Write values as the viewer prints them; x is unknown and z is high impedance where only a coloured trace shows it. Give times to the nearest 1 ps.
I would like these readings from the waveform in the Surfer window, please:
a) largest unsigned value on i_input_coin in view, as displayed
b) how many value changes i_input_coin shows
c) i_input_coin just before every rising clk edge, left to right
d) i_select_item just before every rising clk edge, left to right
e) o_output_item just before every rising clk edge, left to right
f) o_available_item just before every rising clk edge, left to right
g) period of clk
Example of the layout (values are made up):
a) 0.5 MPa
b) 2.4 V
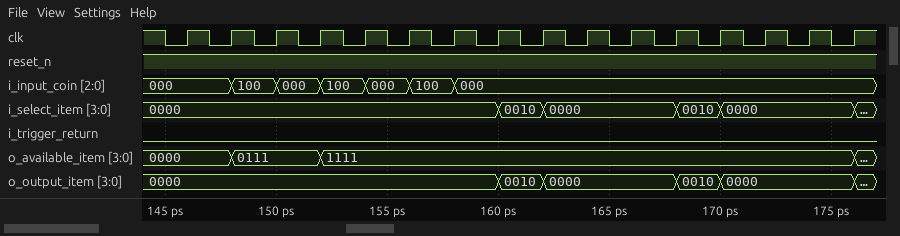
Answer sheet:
a) 100
b) 6
c) 000, 000, 100, 000, 100, 000, 100, 000, 000, 000, 000, 000, 000, 000, 000, 000
d) 0000, 0000, 0000, 0000, 0000, 0000, 0000, 0000, 0010, 0000, 0000, 0000, 0010, 0000, 0000, 0000
e) 0000, 0000, 0000, 0000, 0000, 0000, 0000, 0000, 0010, 0000, 0000, 0000, 0010, 0000, 0000, 0000
f) 0000, 0000, 0111, 0111, 1111, 1111, 1111, 1111, 1111, 1111, 1111, 1111, 1111, 1111, 1111, 1111
g) 2 ps
